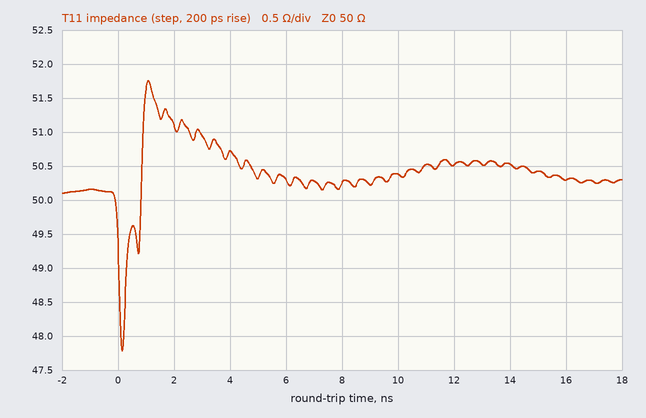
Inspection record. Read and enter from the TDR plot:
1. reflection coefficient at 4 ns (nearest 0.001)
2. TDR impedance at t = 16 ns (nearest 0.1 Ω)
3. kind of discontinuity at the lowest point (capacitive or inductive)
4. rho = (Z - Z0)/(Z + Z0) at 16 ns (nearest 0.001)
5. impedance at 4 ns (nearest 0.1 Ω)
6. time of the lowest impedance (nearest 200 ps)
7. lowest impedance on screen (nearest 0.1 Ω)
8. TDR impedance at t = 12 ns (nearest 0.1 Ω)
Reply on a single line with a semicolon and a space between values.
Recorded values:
+0.007; 50.3 Ω; capacitive; +0.003; 50.7 Ω; 200 ps; 47.8 Ω; 50.5 Ω
